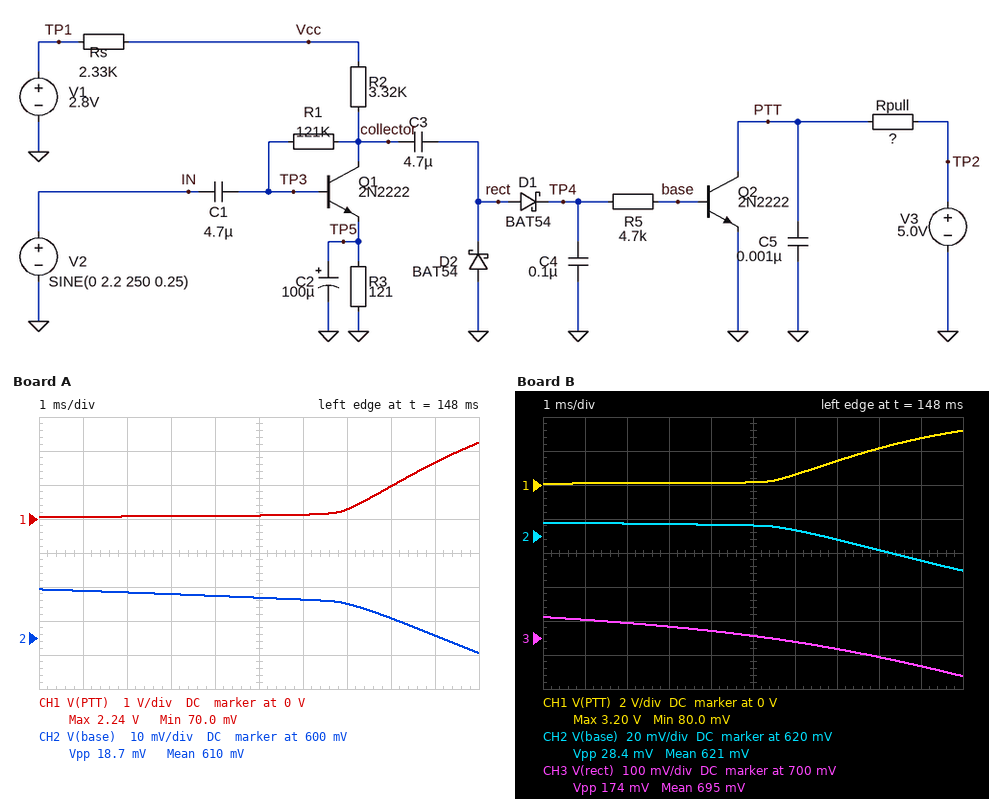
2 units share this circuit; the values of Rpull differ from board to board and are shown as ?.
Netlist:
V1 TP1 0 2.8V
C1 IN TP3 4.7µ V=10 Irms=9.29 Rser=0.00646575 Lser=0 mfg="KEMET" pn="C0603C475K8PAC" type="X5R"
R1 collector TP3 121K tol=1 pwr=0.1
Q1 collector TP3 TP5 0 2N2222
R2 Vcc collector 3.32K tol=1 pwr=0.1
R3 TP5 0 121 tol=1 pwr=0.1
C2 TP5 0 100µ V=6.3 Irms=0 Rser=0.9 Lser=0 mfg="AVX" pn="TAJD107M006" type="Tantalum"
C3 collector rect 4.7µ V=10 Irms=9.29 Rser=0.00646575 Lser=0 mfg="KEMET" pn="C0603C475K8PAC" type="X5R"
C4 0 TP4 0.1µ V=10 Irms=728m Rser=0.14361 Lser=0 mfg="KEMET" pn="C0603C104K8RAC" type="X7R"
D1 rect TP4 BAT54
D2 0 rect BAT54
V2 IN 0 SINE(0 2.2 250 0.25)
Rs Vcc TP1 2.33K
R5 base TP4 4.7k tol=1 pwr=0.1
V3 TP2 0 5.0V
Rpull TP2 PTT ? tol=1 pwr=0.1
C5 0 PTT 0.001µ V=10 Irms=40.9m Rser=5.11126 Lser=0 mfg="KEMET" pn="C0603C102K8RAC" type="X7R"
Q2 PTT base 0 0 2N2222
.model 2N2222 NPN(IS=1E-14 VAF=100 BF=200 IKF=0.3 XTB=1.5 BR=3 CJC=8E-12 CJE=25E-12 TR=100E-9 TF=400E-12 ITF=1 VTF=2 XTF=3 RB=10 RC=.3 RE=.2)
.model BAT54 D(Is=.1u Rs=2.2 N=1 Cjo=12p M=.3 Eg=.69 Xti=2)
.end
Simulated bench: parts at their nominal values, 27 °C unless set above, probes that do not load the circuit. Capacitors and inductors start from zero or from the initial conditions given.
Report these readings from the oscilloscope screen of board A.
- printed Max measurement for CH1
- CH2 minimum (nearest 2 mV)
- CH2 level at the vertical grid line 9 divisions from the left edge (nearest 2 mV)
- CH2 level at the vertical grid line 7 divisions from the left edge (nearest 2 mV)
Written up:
2.24 V
596 mV
600 mV
610 mV
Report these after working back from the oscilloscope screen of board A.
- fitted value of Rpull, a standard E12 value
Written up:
27 kΩ
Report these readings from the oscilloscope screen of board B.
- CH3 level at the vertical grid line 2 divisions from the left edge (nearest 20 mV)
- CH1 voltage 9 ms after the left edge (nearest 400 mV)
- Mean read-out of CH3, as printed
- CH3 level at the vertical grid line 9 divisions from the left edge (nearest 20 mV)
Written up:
740 mV
2.8 V
695 mV
620 mV
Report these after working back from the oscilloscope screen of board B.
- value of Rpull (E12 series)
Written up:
15 kΩ
